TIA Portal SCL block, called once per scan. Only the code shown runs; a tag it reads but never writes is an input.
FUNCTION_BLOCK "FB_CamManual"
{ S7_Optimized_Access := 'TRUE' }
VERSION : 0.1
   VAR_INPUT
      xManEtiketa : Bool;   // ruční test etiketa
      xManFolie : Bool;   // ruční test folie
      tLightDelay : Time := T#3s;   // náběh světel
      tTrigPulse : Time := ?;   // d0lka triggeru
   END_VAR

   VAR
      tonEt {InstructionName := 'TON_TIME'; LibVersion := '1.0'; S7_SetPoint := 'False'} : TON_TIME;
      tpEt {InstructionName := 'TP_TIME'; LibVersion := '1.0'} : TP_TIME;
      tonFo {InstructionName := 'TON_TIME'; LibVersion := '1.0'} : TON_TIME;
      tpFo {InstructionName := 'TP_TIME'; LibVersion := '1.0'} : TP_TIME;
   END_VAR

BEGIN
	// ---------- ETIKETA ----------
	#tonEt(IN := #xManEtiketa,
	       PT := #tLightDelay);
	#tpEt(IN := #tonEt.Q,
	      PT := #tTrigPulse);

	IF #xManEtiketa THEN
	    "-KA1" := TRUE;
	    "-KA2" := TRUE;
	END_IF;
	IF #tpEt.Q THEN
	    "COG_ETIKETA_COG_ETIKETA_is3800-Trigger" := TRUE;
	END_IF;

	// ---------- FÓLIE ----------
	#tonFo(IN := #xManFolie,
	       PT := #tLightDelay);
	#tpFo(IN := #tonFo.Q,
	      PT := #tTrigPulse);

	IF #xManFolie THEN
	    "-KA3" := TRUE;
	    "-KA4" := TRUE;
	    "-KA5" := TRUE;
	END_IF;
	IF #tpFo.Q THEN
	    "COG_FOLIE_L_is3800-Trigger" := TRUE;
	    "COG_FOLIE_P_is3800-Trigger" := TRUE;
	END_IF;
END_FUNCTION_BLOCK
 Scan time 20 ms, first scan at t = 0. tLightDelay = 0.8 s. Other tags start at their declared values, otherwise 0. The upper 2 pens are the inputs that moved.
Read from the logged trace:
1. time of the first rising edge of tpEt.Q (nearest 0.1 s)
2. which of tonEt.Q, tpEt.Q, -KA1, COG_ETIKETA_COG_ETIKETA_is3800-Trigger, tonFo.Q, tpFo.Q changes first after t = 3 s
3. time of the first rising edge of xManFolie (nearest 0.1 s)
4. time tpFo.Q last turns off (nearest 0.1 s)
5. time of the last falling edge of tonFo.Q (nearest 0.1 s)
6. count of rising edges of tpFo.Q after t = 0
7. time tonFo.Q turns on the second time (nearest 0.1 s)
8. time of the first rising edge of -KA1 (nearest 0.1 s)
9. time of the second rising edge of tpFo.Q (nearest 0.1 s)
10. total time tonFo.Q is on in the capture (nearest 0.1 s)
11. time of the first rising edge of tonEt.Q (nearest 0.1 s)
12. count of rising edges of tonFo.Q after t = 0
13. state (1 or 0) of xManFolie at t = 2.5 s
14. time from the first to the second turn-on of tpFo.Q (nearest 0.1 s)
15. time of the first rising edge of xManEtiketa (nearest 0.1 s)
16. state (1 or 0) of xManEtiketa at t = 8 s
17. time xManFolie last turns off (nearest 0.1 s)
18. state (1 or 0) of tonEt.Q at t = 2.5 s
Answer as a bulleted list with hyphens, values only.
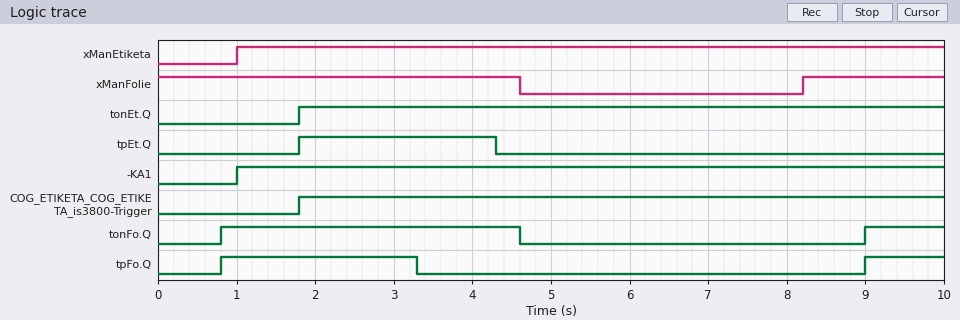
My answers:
- 1.8 s
- tpFo.Q
- 8.2 s
- 3.3 s
- 4.6 s
- 2
- 9.0 s
- 1.0 s
- 9.0 s
- 4.8 s
- 1.8 s
- 2
- 1
- 8.2 s
- 1.0 s
- 1
- 4.6 s
- 1
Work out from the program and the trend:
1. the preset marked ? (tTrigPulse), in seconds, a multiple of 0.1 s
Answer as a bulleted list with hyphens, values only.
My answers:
- 2.5 s
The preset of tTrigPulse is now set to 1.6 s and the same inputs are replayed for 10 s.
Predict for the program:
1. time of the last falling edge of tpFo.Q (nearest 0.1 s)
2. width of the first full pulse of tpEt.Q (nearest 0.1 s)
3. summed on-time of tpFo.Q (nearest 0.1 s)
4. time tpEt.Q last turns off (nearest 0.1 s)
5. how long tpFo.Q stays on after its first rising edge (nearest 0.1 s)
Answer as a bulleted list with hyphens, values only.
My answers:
- 2.4 s
- 1.6 s
- 2.6 s
- 3.4 s
- 1.6 s
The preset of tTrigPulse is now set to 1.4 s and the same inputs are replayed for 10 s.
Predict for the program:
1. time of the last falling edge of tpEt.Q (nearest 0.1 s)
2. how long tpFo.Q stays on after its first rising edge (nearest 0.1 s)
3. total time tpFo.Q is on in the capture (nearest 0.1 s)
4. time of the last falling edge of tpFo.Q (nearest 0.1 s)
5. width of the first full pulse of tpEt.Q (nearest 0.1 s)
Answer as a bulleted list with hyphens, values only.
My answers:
- 3.2 s
- 1.4 s
- 2.4 s
- 2.2 s
- 1.4 s
